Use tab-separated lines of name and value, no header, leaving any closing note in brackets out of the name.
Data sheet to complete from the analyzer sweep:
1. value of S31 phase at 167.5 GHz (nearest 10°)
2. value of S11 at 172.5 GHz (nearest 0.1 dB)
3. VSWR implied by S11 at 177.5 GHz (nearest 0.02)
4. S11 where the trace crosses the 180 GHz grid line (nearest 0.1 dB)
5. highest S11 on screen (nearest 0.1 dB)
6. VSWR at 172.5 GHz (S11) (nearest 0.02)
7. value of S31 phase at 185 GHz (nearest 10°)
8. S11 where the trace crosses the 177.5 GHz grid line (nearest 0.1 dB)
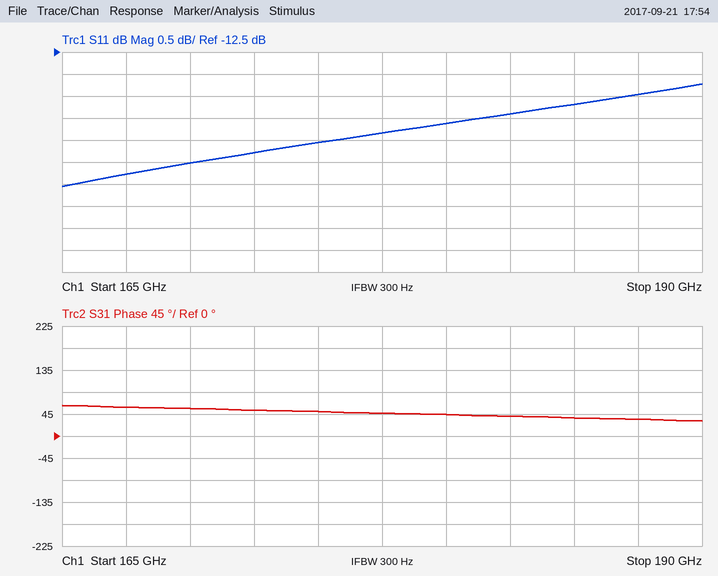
value of S31 phase at 167.5 GHz	60°
value of S11 at 172.5 GHz	-14.8 dB
VSWR implied by S11 at 177.5 GHz	1.48
S11 where the trace crosses the 180 GHz grid line	-14.1 dB
highest S11 on screen	-13.2 dB
VSWR at 172.5 GHz (S11)	1.44
value of S31 phase at 185 GHz	40°
S11 where the trace crosses the 177.5 GHz grid line	-14.3 dB
